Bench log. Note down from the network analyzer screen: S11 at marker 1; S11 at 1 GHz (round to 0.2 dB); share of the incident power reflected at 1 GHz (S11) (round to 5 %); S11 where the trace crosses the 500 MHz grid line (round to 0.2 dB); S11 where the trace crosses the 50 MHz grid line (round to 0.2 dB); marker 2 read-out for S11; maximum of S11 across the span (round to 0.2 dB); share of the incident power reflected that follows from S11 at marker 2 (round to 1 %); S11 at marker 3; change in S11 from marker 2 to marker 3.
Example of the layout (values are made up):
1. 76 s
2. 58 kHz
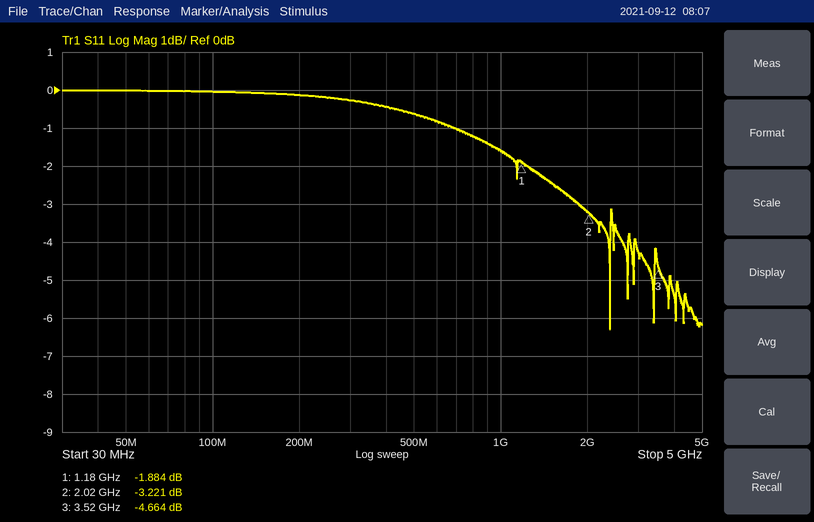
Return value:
1. -1.884 dB
2. -1.6 dB
3. 70 %
4. -0.6 dB
5. 0.0 dB
6. -3.221 dB
7. 0.0 dB
8. 48 %
9. -4.664 dB
10. -1.443 dB
